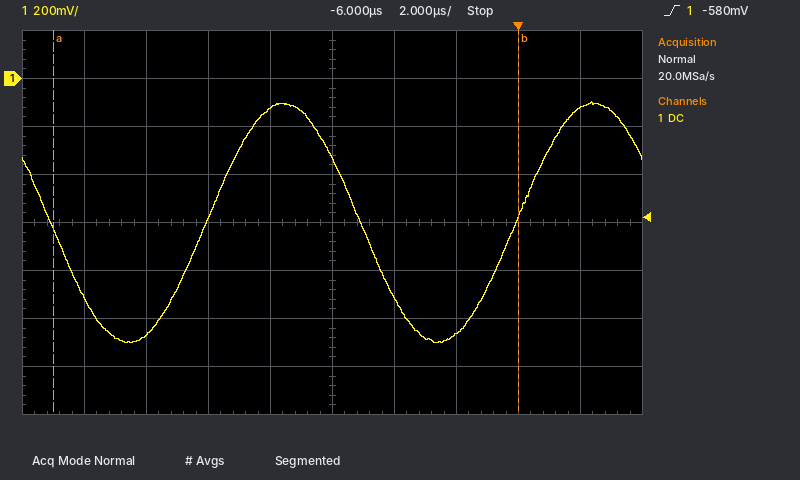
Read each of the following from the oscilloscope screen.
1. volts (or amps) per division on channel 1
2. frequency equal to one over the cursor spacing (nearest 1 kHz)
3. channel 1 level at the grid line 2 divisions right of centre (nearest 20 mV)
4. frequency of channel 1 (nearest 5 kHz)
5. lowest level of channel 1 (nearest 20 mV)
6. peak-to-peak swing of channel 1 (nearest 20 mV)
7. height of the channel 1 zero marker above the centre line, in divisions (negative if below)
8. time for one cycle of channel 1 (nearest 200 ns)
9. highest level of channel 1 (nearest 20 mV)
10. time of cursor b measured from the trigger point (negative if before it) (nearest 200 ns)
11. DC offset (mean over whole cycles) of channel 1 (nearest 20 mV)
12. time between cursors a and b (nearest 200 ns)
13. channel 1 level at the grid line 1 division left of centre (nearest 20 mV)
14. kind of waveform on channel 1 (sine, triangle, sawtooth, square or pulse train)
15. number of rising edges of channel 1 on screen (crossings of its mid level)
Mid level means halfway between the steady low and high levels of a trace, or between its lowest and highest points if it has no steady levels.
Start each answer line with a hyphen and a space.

- 200 mV
- 67 kHz
- -1.06 V
- 100 kHz
- -1.10 V
- 1.00 V
- +3.0 div
- 10.0 µs
- -100 mV
- 0.0 µs
- -600 mV
- 15.0 µs
- -120 mV
- sine
- 2
